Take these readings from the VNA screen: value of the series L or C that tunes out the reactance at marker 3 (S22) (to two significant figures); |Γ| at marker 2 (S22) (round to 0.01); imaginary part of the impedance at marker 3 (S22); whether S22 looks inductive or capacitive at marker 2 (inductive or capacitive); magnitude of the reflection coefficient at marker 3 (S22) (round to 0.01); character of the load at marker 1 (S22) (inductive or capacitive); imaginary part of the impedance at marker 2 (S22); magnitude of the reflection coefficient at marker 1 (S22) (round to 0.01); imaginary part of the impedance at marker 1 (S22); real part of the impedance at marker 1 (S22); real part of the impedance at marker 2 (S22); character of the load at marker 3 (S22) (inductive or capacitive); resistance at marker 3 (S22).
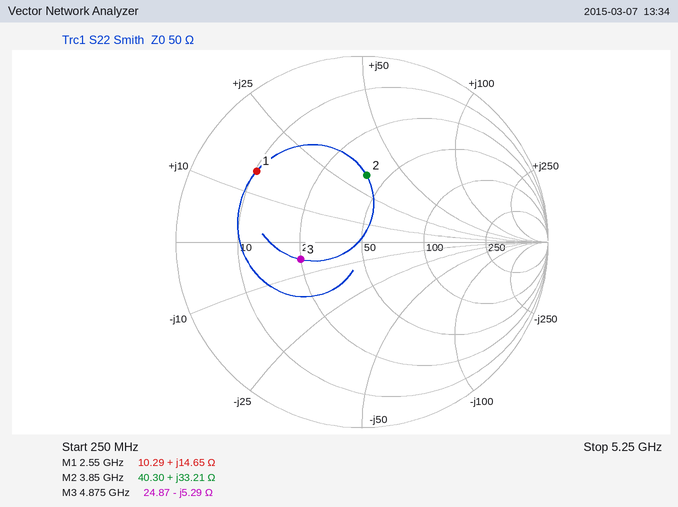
170 pH
0.36
-5.29 Ω
inductive
0.34
inductive
+33.21 Ω
0.68
+14.65 Ω
10.29 Ω
40.30 Ω
capacitive
24.87 Ω
